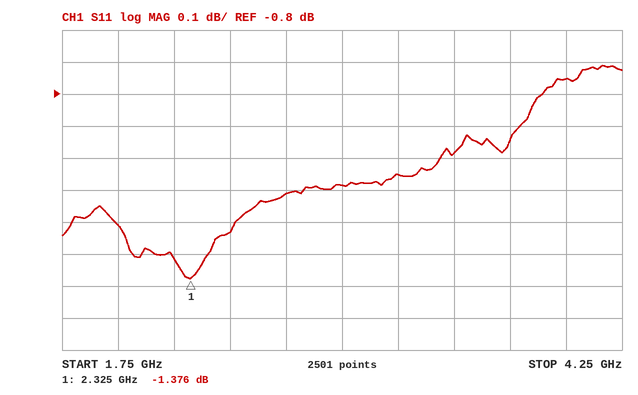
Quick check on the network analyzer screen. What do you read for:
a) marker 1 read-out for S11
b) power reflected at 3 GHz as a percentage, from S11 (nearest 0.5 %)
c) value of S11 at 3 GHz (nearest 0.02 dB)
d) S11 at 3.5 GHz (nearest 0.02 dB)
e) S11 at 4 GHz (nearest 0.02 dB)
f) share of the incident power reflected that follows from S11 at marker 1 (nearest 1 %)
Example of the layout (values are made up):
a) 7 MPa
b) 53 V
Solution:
a) -1.376 dB
b) 78.0 %
c) -1.08 dB
d) -0.98 dB
e) -0.76 dB
f) 73 %
